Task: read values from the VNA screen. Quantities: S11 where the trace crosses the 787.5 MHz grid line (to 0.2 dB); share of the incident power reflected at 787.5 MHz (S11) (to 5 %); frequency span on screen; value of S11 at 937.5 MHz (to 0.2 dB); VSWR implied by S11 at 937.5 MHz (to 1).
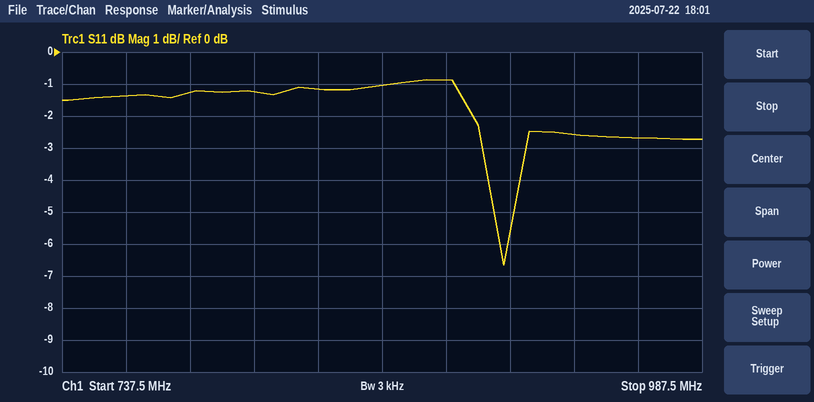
-1.2 dB
75 %
250 MHz
-2.6 dB
7
